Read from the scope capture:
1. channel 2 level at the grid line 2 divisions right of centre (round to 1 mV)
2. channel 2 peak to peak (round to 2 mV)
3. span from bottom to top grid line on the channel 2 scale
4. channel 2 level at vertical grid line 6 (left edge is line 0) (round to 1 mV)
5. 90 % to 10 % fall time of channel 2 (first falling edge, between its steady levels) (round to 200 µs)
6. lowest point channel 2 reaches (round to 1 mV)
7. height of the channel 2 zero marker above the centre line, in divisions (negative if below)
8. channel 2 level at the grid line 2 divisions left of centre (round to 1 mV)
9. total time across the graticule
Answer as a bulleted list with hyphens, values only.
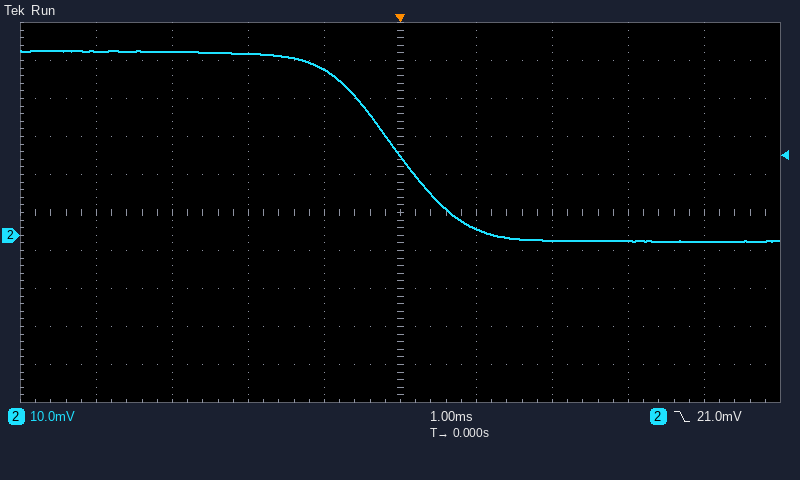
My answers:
- -1 mV
- 50 mV
- 100 mV
- 2 mV
- 1.8 ms
- -2 mV
- -0.6 div
- 48 mV
- 10 ms
